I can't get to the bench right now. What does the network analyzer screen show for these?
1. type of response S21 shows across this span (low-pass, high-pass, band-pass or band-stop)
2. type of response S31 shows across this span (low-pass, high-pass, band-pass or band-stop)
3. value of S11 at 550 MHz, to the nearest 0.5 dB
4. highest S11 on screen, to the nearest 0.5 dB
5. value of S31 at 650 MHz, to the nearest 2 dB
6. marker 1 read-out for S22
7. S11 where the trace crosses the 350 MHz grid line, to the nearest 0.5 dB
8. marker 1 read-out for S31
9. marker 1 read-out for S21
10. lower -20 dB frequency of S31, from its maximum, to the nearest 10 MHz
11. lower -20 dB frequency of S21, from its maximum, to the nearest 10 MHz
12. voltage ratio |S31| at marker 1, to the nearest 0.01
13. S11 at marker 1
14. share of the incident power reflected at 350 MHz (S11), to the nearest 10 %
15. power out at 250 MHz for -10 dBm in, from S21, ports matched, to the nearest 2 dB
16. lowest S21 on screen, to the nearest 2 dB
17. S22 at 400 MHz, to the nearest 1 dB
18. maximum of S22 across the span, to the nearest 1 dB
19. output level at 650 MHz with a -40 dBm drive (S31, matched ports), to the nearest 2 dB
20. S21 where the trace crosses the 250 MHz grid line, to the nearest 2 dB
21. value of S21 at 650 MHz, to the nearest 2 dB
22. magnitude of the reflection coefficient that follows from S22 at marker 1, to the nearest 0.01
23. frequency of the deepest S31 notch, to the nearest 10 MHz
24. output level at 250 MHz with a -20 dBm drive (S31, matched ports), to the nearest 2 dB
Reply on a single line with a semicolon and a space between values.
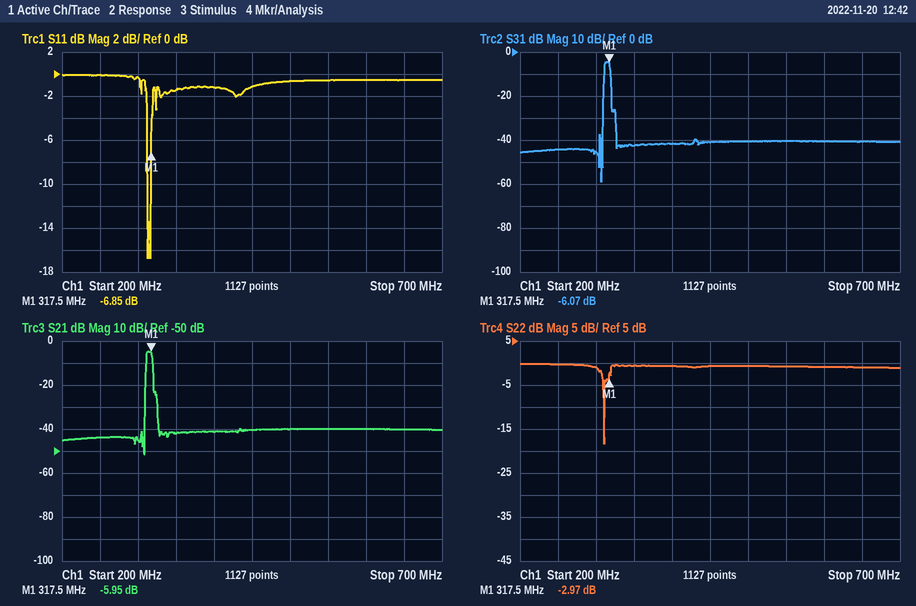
band-pass; band-pass; -0.5 dB; 0.0 dB; -40 dB; -2.97 dB; -1.5 dB; -6.07 dB; -5.95 dB; 310 MHz; 310 MHz; 0.50; -6.85 dB; 70 %; -54 dBm; -52 dB; -1 dB; 0 dB; -80 dBm; -44 dB; -40 dB; 0.71; 310 MHz; -64 dBm
